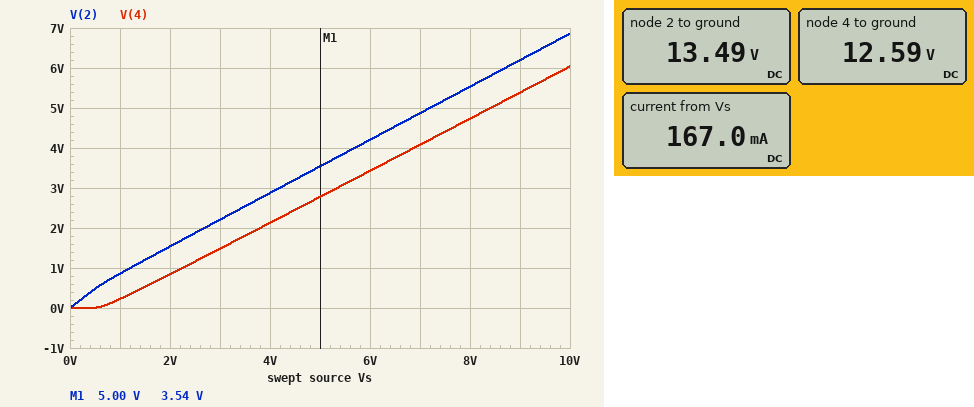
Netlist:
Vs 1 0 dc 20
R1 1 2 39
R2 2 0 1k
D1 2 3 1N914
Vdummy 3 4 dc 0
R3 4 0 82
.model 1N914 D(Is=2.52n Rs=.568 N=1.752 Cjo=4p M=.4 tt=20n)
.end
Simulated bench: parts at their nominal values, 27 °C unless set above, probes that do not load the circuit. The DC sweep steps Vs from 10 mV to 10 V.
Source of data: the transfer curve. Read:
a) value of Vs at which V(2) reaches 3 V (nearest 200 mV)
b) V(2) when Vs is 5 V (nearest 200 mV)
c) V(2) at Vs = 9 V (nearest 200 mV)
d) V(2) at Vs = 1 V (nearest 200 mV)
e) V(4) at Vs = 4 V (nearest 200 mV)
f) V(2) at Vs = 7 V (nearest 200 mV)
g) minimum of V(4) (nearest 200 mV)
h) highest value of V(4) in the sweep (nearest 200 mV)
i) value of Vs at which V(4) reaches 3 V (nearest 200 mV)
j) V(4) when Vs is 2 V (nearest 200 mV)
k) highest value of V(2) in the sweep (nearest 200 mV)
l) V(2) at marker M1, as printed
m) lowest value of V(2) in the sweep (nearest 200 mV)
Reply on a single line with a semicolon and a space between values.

4.2 V; 3.6 V; 6.2 V; 800 mV; 2.2 V; 4.8 V; 0 V; 6.0 V; 5.4 V; 800 mV; 6.8 V; 3.54 V; 0 V
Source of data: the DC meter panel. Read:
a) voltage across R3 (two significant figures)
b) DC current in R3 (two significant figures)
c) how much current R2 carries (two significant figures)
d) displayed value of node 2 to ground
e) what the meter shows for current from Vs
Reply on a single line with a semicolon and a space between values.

13 V; 150 mA; 13 mA; 13.49 V; 167.0 mA
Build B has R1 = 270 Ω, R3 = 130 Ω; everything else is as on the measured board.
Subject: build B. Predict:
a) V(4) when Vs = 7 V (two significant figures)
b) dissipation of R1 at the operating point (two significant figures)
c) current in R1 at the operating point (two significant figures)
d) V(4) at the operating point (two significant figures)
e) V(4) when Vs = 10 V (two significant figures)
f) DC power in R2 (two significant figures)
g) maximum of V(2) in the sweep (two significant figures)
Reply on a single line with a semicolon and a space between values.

1.8 V; 680 mW; 50 mA; 5.7 V; 2.7 V; 42 mW; 3.4 V
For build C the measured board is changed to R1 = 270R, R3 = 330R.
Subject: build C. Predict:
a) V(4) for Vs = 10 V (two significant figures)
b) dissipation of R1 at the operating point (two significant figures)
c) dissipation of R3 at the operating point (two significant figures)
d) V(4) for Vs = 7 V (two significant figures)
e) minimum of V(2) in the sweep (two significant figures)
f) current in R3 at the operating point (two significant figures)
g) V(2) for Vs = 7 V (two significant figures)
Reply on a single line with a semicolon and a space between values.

4.4 V; 380 mW; 250 mW; 2.9 V; 7.9 mV; 28 mA; 3.6 V
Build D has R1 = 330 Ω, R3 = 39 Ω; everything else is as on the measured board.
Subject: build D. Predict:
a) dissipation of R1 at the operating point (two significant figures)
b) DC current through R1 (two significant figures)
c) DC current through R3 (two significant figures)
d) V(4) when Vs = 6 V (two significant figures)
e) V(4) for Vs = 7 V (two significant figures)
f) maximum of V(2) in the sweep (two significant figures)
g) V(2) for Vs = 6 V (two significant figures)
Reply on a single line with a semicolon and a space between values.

900 mW; 52 mA; 50 mA; 520 mV; 620 mV; 1.7 V; 1.2 V
